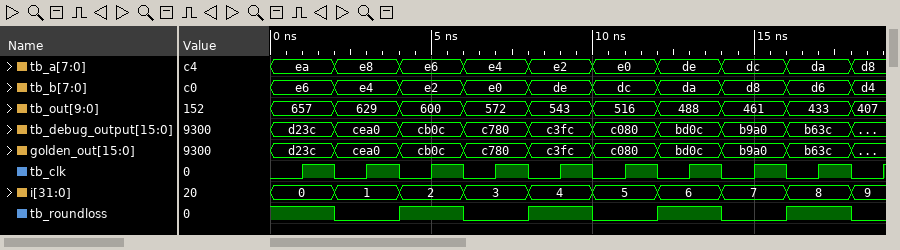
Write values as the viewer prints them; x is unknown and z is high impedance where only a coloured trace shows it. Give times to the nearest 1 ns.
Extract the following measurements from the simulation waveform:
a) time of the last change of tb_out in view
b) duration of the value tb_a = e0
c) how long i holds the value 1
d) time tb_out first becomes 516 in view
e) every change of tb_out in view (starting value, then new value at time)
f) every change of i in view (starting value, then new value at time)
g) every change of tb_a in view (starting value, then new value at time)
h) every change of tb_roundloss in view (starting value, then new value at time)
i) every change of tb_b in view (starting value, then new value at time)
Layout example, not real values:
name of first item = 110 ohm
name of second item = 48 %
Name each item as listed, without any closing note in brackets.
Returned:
time of the last change of tb_out in view = 18 ns
duration of the value tb_a = e0 = 2 ns
how long i holds the value 1 = 2 ns
time tb_out first becomes 516 in view = 10 ns
every change of tb_out in view = 657, 629 at 2 ns, 600 at 4 ns, 572 at 6 ns, 543 at 8 ns, 516 at 10 ns, 488 at 12 ns, 461 at 14 ns, 433 at 16 ns, 407 at 18 ns
every change of i in view = 0, 1 at 2 ns, 2 at 4 ns, 3 at 6 ns, 4 at 8 ns, 5 at 10 ns, 6 at 12 ns, 7 at 14 ns, 8 at 16 ns, 9 at 18 ns
every change of tb_a in view = ea, e8 at 2 ns, e6 at 4 ns, e4 at 6 ns, e2 at 8 ns, e0 at 10 ns, de at 12 ns, dc at 14 ns, da at 16 ns, d8 at 18 ns
every change of tb_roundloss in view = 1, 0 at 2 ns, 1 at 4 ns, 0 at 6 ns, 1 at 8 ns, 0 at 10 ns, 1 at 12 ns, 0 at 14 ns, 1 at 16 ns, 0 at 18 ns
every change of tb_b in view = e6, e4 at 2 ns, e2 at 4 ns, e0 at 6 ns, de at 8 ns, dc at 10 ns, da at 12 ns, d8 at 14 ns, d6 at 16 ns, d4 at 18 ns
